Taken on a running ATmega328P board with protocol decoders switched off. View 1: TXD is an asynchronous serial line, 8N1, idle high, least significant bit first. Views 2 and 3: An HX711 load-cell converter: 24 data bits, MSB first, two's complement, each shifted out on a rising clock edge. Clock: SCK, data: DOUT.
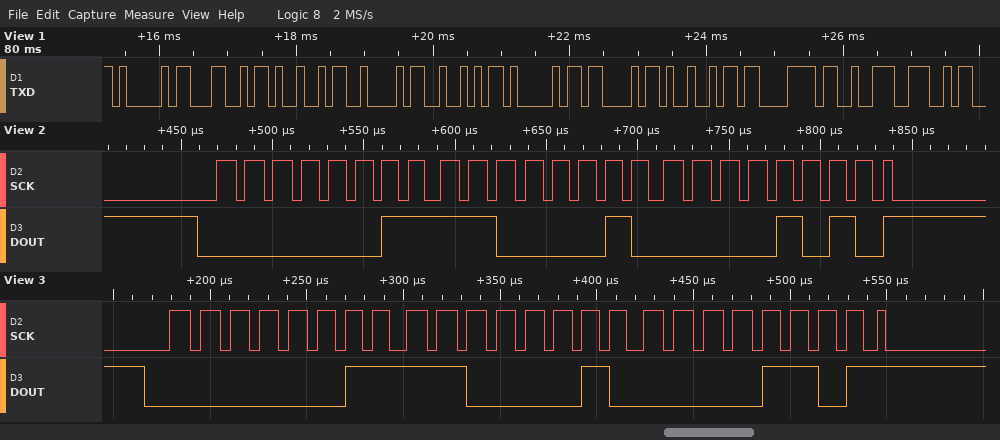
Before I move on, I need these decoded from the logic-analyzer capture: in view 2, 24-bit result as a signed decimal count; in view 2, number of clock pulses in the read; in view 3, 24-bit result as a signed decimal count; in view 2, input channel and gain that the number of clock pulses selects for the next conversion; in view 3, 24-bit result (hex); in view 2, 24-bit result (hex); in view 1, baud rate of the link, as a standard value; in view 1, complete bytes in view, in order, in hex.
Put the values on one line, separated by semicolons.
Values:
246282; 25; 246285; channel A, gain 128; 0x03C20D; 0x03C20A; 9600 baud; 41 4C 49 42 52 41 43 49 C3 93 4E
